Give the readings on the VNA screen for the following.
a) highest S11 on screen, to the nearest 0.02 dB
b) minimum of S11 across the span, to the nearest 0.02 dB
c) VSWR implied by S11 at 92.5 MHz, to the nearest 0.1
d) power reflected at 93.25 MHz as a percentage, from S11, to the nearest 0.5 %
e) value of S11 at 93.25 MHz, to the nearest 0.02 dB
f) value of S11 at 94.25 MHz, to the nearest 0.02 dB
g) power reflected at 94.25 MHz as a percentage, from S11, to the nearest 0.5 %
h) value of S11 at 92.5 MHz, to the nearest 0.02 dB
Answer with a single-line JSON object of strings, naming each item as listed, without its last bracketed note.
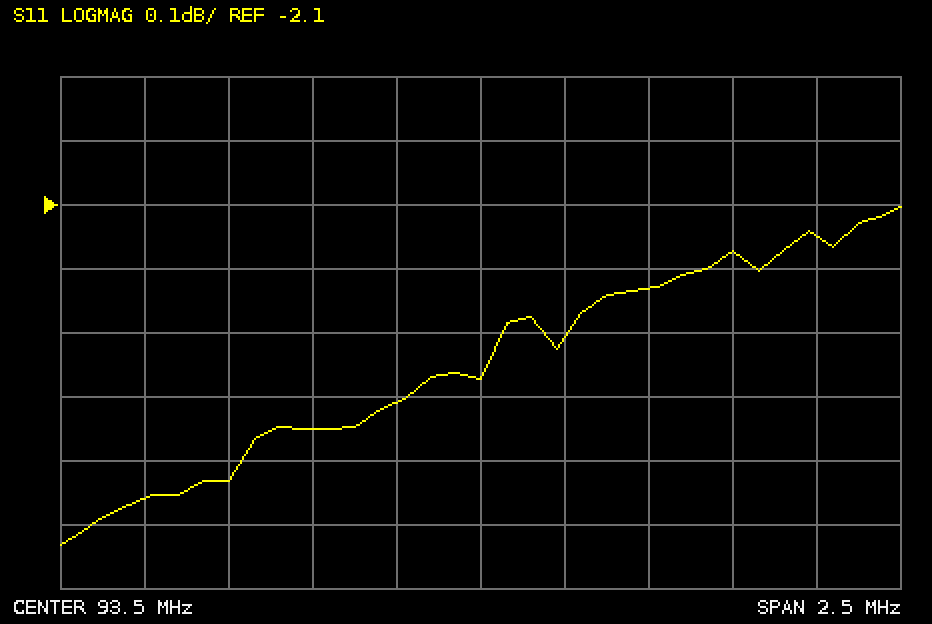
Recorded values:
{"highest S11 on screen, to the nearest 0.02 dB": "-2.10 dB", "minimum of S11 across the span, to the nearest 0.02 dB": "-2.64 dB", "VSWR implied by S11 at 92.5 MHz, to the nearest 0.1": "6.8", "power reflected at 93.25 MHz as a percentage, from S11, to the nearest 0.5 %": "57.5 %", "value of S11 at 93.25 MHz, to the nearest 0.02 dB": "-2.40 dB", "value of S11 at 94.25 MHz, to the nearest 0.02 dB": "-2.18 dB", "power reflected at 94.25 MHz as a percentage, from S11, to the nearest 0.5 %": "60.5 %", "value of S11 at 92.5 MHz, to the nearest 0.02 dB": "-2.56 dB"}
